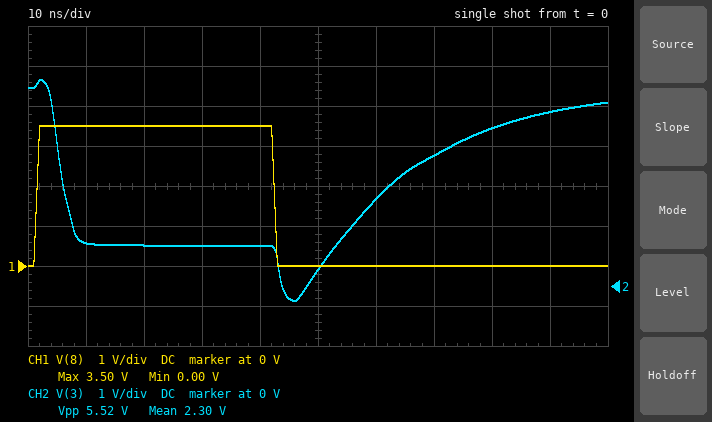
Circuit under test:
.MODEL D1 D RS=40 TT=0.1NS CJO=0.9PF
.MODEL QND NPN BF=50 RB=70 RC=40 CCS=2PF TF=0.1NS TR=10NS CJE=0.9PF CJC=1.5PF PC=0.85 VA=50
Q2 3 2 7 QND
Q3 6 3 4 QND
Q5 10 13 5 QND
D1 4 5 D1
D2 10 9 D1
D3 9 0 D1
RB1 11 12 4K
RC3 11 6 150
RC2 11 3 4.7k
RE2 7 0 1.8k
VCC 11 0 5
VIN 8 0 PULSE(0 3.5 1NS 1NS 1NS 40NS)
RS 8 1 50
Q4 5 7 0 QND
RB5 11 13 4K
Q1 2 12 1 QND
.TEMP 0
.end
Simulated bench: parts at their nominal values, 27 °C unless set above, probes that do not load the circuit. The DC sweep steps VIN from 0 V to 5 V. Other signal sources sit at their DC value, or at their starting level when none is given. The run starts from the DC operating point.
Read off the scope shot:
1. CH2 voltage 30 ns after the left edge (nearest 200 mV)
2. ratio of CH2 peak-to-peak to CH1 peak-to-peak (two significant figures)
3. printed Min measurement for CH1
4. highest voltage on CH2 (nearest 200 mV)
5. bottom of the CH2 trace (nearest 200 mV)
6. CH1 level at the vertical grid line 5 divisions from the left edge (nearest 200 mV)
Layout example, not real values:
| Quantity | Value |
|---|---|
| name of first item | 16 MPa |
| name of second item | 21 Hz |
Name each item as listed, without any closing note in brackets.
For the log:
| Quantity | Value |
|---|---|
| CH2 voltage 30 ns after the left edge | 1.0 V |
| ratio of CH2 peak-to-peak to CH1 peak-to-peak | 1.6 |
| printed Min measurement for CH1 | 0.00 V |
| highest voltage on CH2 | 5.2 V |
| bottom of the CH2 trace | -400 mV |
| CH1 level at the vertical grid line 5 divisions from the left edge | 0 V |
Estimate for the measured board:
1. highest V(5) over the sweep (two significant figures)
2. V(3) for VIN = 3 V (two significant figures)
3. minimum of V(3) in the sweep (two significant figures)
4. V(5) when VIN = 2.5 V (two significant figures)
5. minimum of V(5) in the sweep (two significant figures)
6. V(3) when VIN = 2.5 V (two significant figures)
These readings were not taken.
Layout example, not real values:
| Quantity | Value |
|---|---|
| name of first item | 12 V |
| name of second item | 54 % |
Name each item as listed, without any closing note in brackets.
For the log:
| Quantity | Value |
|---|---|
| highest V(5) over the sweep | 3.4 V |
| V(3) for VIN = 3 V | 1.0 V |
| minimum of V(3) in the sweep | 950 mV |
| V(5) when VIN = 2.5 V | 64 mV |
| minimum of V(5) in the sweep | 64 mV |
| V(3) when VIN = 2.5 V | 1.0 V |
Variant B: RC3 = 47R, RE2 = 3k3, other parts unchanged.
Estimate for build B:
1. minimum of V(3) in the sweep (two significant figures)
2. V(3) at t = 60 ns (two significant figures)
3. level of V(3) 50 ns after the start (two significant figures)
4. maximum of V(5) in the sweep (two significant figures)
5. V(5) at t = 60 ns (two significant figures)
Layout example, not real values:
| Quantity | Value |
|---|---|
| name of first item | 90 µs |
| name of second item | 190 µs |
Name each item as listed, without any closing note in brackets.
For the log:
| Quantity | Value |
|---|---|
| minimum of V(3) in the sweep | 970 mV |
| V(3) at t = 60 ns | 2.0 V |
| level of V(3) 50 ns after the start | 410 mV |
| maximum of V(5) in the sweep | 3.4 V |
| V(5) at t = 60 ns | 310 mV |
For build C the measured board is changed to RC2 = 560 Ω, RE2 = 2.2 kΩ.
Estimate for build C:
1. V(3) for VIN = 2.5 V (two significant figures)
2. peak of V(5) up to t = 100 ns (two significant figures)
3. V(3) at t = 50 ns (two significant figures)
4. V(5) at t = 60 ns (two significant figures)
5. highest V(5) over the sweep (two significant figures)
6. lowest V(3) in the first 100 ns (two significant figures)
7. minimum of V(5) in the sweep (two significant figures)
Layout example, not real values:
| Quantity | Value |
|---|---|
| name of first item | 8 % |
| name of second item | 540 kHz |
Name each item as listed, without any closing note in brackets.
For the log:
| Quantity | Value |
|---|---|
| V(3) for VIN = 2.5 V | 1.6 V |
| peak of V(5) up to t = 100 ns | 3.9 V |
| V(3) at t = 50 ns | 3.3 V |
| V(5) at t = 60 ns | 800 mV |
| highest V(5) over the sweep | 3.5 V |
| lowest V(3) in the first 100 ns | 1.0 V |
| minimum of V(5) in the sweep | 85 mV |
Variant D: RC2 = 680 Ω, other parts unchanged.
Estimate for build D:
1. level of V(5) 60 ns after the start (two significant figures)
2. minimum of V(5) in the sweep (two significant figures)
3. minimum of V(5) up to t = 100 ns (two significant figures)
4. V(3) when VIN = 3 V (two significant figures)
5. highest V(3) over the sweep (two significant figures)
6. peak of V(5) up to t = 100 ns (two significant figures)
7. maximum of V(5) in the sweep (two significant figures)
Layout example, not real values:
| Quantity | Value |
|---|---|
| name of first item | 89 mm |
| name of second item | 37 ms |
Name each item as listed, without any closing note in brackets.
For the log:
| Quantity | Value |
|---|---|
| level of V(5) 60 ns after the start | 800 mV |
| minimum of V(5) in the sweep | 65 mV |
| minimum of V(5) up to t = 100 ns | 27 mV |
| V(3) when VIN = 3 V | 1.5 V |
| highest V(3) over the sweep | 5.0 V |
| peak of V(5) up to t = 100 ns | 3.9 V |
| maximum of V(5) in the sweep | 3.5 V |
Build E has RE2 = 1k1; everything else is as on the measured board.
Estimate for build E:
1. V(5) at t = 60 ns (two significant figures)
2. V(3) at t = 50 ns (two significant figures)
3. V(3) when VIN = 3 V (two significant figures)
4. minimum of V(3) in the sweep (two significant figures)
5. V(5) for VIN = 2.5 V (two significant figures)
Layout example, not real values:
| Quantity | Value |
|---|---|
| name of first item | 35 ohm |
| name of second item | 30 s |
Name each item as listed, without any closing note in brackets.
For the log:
| Quantity | Value |
|---|---|
| V(5) at t = 60 ns | 1.3 V |
| V(3) at t = 50 ns | 380 mV |
| V(3) when VIN = 3 V | 980 mV |
| minimum of V(3) in the sweep | 920 mV |
| V(5) for VIN = 2.5 V | 66 mV |
